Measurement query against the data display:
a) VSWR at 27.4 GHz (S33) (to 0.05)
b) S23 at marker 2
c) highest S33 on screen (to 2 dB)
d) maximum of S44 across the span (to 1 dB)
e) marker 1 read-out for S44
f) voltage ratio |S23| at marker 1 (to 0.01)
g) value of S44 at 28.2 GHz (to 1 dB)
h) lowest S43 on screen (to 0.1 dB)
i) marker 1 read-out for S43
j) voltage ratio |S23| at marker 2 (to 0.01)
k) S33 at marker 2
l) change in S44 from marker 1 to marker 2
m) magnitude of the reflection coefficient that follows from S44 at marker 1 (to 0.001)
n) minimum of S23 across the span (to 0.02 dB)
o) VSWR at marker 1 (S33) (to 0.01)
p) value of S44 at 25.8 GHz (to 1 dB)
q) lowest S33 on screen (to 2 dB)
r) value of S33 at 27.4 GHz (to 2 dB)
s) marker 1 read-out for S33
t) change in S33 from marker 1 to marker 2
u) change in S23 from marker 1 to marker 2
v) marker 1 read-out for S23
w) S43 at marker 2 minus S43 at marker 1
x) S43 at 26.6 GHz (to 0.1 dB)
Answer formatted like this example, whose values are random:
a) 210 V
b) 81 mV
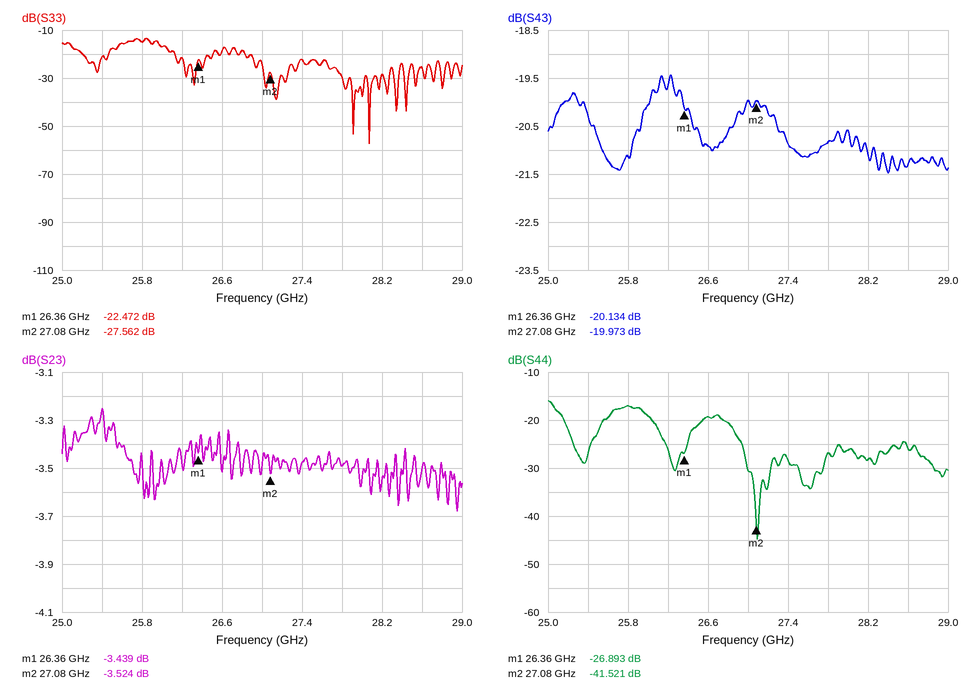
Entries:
a) 1.15
b) -3.524 dB
c) -14 dB
d) -16 dB
e) -26.893 dB
f) 0.67
g) -28 dB
h) -21.5 dB
i) -20.134 dB
j) 0.67
k) -27.562 dB
l) -14.628 dB
m) 0.045
n) -3.68 dB
o) 1.16
p) -17 dB
q) -58 dB
r) -22 dB
s) -22.472 dB
t) -5.090 dB
u) -0.085 dB
v) -3.439 dB
w) 0.161 dB
x) -20.9 dB
